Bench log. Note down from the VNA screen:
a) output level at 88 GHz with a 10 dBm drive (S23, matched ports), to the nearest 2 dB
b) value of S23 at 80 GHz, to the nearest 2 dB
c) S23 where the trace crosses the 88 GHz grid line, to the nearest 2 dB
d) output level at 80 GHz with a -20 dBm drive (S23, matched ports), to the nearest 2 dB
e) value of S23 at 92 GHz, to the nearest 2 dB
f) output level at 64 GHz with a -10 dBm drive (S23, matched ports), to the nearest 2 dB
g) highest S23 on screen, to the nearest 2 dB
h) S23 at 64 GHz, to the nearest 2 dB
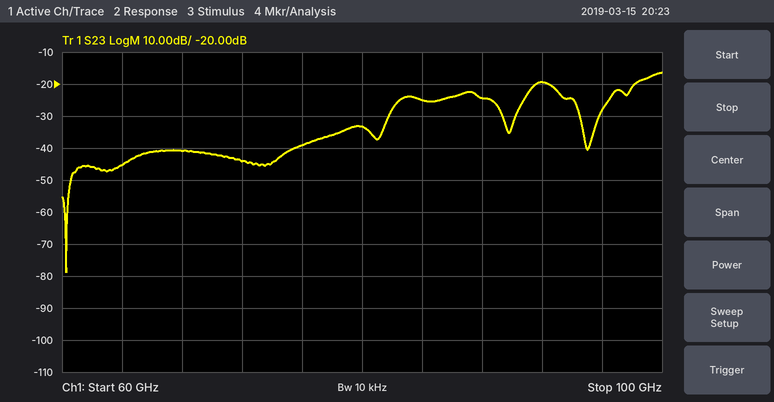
-14 dBm
-34 dB
-24 dB
-54 dBm
-20 dB
-56 dBm
-16 dB
-46 dB
